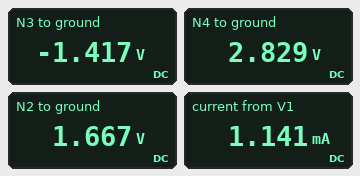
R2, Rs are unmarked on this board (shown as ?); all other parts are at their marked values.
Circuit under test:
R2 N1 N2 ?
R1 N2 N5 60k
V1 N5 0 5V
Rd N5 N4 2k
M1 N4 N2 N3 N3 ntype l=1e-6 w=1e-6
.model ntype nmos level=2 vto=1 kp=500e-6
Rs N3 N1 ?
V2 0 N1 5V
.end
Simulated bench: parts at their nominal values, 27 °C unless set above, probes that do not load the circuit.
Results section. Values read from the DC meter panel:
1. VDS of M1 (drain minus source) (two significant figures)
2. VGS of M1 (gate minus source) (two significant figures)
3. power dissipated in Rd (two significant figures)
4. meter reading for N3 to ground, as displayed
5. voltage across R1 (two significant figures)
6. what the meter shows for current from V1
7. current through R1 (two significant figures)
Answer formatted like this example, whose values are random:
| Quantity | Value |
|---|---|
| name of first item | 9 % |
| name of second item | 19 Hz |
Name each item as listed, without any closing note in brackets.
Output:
| Quantity | Value |
|---|---|
| VDS of M1 (drain minus source) | 4.2 V |
| VGS of M1 (gate minus source) | 3.1 V |
| power dissipated in Rd | 2.4 mW |
| meter reading for N3 to ground, as displayed | -1.417 V |
| voltage across R1 | 3.3 V |
| what the meter shows for current from V1 | 1.141 mA |
| current through R1 | 56 µA |
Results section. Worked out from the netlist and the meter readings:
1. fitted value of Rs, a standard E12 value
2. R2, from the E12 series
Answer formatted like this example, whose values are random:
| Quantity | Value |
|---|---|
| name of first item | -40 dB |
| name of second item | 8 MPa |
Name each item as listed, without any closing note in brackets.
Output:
| Quantity | Value |
|---|---|
| fitted value of Rs, a standard E12 value | 3.3 kΩ |
| R2, from the E12 series | 120 kΩ |
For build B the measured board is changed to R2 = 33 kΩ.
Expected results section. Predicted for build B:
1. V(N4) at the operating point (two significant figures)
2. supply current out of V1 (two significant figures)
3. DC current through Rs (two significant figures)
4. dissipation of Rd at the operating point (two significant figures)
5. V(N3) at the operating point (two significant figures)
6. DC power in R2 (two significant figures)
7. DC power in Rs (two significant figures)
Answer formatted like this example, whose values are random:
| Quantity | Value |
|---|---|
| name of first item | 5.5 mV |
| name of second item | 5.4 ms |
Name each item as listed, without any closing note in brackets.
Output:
| Quantity | Value |
|---|---|
| V(N4) at the operating point | 4.2 V |
| supply current out of V1 | 500 µA |
| DC current through Rs | 390 µA |
| dissipation of Rd at the operating point | 310 µW |
| V(N3) at the operating point | -3.7 V |
| DC power in R2 | 380 µW |
| DC power in Rs | 510 µW |
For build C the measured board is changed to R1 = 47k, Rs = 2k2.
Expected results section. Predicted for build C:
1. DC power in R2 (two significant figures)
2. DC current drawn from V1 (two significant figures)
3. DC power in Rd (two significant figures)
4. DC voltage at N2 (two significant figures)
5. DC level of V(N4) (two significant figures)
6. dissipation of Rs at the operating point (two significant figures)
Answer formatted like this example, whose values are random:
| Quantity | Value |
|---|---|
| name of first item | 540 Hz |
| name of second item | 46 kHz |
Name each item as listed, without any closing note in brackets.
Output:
| Quantity | Value |
|---|---|
| DC power in R2 | 430 µW |
| DC current drawn from V1 | 1.7 mA |
| DC power in Rd | 5.4 mW |
| DC voltage at N2 | 2.2 V |
| DC level of V(N4) | 1.7 V |
| dissipation of Rs at the operating point | 6.0 mW |
